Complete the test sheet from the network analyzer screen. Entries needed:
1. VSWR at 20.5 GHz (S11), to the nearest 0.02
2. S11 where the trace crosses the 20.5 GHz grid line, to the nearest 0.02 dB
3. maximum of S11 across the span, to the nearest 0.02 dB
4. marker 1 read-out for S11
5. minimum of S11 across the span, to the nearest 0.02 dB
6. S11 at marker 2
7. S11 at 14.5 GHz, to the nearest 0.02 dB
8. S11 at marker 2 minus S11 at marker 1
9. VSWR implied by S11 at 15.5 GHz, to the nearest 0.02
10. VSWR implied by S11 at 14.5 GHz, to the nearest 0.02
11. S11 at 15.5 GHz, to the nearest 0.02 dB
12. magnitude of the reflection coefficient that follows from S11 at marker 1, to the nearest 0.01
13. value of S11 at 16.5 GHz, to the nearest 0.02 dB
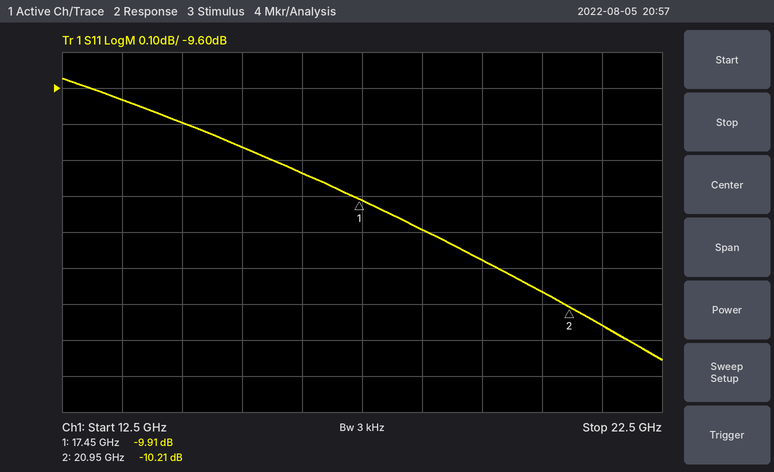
1.90
-10.16 dB
-9.58 dB
-9.91 dB
-10.36 dB
-10.21 dB
-9.70 dB
-0.30 dB
1.96
1.98
-9.76 dB
0.32
-9.84 dB
